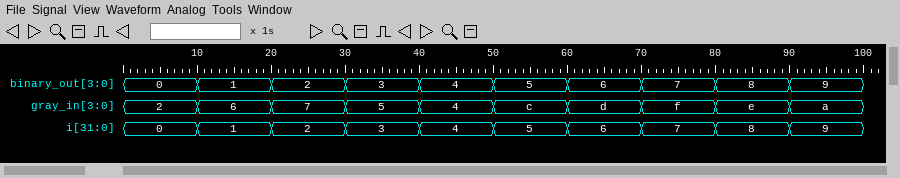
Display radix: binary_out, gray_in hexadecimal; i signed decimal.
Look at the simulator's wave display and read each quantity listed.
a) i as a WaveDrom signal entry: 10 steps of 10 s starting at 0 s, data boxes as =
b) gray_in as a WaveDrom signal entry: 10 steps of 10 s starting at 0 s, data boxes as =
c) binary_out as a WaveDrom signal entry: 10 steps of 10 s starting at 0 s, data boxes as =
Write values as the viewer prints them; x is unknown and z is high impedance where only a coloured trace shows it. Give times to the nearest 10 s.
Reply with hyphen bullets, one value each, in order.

- {name: 'i', wave: '==========', data: '0 1 2 3 4 5 6 7 8 9'}
- {name: 'gray_in', wave: '==========', data: '2 6 7 5 4 c d f e a'}
- {name: 'binary_out', wave: '==========', data: '0 1 2 3 4 5 6 7 8 9'}
